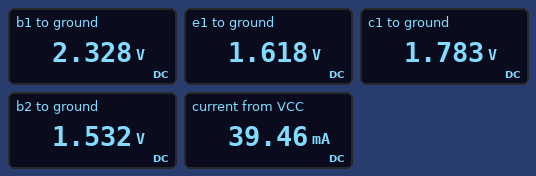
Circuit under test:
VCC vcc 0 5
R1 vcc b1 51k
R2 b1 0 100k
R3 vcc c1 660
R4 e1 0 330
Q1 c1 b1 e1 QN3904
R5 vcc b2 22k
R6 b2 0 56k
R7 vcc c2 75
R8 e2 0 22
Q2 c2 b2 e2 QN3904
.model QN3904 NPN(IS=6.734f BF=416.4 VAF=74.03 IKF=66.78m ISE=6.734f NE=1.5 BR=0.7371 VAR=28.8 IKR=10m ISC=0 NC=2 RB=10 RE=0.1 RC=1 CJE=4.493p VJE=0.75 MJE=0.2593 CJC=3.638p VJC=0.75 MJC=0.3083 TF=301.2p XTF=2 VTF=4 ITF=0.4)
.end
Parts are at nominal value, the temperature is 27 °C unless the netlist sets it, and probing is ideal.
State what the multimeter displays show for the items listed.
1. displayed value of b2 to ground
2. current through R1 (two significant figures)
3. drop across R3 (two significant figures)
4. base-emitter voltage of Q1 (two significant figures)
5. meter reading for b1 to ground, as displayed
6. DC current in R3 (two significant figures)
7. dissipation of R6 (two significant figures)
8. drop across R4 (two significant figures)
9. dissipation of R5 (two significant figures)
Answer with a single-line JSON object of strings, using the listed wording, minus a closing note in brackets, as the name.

{"displayed value of b2 to ground": "1.532 V", "current through R1": "52 µA", "drop across R3": "3.2 V", "base-emitter voltage of Q1": "710 mV", "meter reading for b1 to ground, as displayed": "2.328 V", "DC current in R3": "4.9 mA", "dissipation of R6": "42 µW", "drop across R4": "1.6 V", "dissipation of R5": "550 µW"}
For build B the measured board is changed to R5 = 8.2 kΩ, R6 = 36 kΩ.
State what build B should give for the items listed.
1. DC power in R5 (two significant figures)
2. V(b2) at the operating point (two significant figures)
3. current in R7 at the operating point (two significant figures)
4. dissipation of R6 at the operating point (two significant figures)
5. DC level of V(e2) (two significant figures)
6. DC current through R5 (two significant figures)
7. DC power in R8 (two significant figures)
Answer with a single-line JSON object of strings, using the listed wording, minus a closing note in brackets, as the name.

{"DC power in R5": "1.2 mW", "V(b2) at the operating point": "1.9 V", "current in R7 at the operating point": "49 mA", "dissipation of R6 at the operating point": "98 µW", "DC level of V(e2)": "1.1 V", "DC current through R5": "380 µA", "DC power in R8": "54 mW"}
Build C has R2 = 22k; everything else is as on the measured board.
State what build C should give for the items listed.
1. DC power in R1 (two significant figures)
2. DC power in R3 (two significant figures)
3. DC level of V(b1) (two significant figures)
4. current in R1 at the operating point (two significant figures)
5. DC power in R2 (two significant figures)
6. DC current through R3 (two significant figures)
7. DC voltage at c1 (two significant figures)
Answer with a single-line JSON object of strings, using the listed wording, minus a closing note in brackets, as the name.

{"DC power in R1": "250 µW", "DC power in R3": "3.2 mW", "DC level of V(b1)": "1.4 V", "current in R1 at the operating point": "70 µA", "DC power in R2": "91 µW", "DC current through R3": "2.2 mA", "DC voltage at c1": "3.5 V"}
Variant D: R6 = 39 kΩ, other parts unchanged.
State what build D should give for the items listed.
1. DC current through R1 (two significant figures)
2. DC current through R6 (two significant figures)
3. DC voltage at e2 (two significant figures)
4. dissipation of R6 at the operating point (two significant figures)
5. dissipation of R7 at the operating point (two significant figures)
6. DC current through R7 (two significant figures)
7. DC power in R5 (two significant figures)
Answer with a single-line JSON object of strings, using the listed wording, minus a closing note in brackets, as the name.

{"DC current through R1": "52 µA", "DC current through R6": "38 µA", "DC voltage at e2": "720 mV", "dissipation of R6 at the operating point": "57 µW", "dissipation of R7 at the operating point": "80 mW", "DC current through R7": "33 mA", "DC power in R5": "560 µW"}
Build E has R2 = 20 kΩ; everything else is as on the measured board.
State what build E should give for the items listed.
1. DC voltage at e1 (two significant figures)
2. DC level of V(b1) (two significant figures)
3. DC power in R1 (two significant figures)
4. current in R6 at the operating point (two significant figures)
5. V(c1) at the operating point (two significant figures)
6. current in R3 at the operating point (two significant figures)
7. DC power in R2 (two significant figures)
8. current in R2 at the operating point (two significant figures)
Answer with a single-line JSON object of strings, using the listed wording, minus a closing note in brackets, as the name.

{"DC voltage at e1": "650 mV", "DC level of V(b1)": "1.3 V", "DC power in R1": "260 µW", "current in R6 at the operating point": "27 µA", "V(c1) at the operating point": "3.7 V", "current in R3 at the operating point": "2.0 mA", "DC power in R2": "89 µW", "current in R2 at the operating point": "67 µA"}
